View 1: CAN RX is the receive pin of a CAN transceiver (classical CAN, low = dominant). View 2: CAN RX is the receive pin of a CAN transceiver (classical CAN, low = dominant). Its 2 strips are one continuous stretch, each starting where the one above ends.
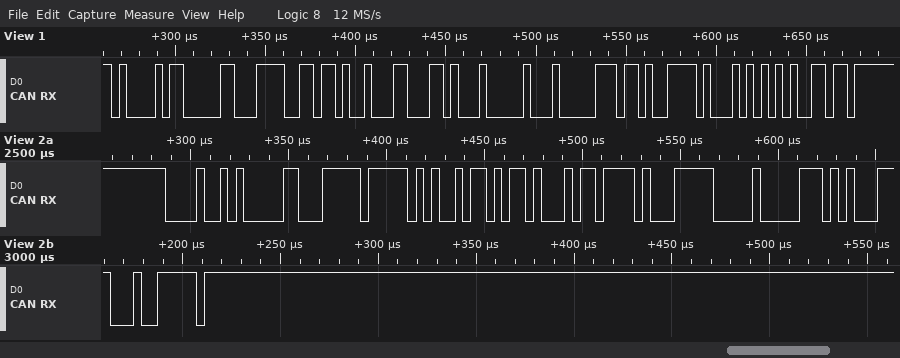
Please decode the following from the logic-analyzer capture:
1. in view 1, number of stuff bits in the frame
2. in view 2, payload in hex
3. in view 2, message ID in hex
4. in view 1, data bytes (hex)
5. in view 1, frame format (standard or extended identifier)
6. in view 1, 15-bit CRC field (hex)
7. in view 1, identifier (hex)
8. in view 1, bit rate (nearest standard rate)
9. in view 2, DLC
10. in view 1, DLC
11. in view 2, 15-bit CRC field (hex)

3
FF E9 6B 45 BD 1F 00 6A
0x094
F3 69 18 D1 00 83 69 E8
standard
0x554D
0x42C
250 kbit/s
8
8
0x1C4F
